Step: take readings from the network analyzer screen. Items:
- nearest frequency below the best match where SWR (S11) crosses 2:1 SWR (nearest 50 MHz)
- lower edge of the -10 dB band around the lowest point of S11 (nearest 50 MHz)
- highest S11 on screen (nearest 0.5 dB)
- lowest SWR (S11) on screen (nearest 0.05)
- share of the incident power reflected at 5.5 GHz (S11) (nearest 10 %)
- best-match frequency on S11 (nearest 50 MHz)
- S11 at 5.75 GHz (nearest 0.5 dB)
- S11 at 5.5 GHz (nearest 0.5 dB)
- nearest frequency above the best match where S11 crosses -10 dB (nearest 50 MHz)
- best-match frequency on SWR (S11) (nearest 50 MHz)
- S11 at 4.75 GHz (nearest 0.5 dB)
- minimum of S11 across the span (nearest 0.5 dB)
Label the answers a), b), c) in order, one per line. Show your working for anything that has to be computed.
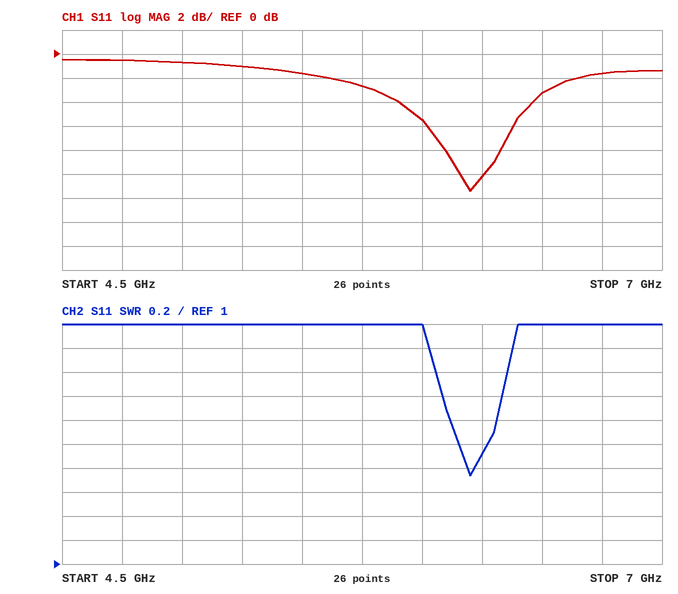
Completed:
a) 6.15 GHz
b) 6.15 GHz
c) -0.5 dB
d) 1.75
e) 10^(-1.5/10) ≈ 70.8 %, so 70 % to the nearest 10 %
f) 6.20 GHz
g) -2.5 dB
h) -1.5 dB
i) 6.25 GHz
j) 6.20 GHz
k) -0.5 dB
l) -11.5 dB
